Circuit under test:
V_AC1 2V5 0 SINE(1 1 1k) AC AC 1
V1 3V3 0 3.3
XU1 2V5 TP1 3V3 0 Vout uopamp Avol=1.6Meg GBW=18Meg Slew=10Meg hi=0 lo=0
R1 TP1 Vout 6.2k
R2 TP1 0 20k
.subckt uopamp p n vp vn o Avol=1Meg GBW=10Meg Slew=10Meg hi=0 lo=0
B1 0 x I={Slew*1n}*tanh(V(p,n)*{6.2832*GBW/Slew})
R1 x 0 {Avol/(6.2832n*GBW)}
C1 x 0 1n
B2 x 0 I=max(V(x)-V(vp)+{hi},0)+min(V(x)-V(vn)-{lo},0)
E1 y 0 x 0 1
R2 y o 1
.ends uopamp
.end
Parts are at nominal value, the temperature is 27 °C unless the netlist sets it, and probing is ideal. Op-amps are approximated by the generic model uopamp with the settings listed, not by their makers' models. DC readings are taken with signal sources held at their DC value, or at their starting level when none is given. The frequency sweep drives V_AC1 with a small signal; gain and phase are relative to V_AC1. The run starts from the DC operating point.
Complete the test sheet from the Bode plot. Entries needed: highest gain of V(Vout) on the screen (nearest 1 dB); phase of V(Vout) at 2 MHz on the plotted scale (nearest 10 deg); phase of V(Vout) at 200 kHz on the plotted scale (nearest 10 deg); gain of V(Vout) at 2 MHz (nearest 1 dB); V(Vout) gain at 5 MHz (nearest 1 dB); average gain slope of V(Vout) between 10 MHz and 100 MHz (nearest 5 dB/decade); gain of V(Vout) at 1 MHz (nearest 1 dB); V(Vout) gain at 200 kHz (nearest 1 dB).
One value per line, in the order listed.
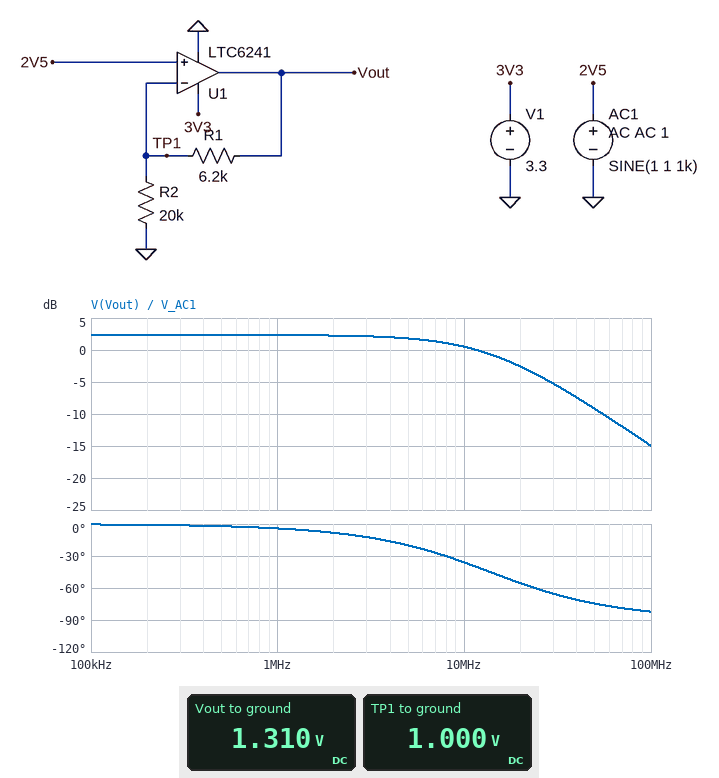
2 dB
-10 deg
0 deg
2 dB
2 dB
-15 dB/decade
2 dB
2 dB
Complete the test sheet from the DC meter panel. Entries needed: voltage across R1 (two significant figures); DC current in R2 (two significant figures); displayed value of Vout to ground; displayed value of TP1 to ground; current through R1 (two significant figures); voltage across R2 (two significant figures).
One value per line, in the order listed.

310 mV
50 µA
1.310 V
1.000 V
50 µA
1.0 V
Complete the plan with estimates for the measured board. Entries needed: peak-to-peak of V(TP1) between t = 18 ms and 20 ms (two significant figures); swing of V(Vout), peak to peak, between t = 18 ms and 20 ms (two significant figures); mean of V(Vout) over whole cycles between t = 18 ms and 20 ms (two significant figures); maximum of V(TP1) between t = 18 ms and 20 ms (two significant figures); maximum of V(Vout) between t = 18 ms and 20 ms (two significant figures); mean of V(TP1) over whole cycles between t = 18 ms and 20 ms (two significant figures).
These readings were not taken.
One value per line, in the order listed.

2.0 V
2.6 V
1.3 V
2.0 V
2.6 V
1.0 V
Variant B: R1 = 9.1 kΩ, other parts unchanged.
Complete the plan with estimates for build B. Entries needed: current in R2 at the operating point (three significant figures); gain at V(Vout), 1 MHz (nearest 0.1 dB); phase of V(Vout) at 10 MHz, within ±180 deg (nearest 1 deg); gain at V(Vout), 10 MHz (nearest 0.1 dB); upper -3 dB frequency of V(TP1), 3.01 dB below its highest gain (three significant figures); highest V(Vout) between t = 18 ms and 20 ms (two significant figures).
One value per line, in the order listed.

50.0 µA
3.2 dB
-39 deg
1.1 dB
12.4 MHz
2.9 V
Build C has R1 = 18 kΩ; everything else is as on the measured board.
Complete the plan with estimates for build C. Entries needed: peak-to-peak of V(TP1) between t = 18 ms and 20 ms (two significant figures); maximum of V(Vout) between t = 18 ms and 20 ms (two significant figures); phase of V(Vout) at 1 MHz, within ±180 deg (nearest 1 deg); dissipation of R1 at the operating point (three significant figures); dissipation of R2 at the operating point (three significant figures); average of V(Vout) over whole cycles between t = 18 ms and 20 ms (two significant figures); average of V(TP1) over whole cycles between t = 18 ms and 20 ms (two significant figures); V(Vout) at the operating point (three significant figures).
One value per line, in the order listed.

1.7 V
3.3 V
-6 deg
45.0 µW
50.0 µW
1.8 V
960 mV
1.90 V
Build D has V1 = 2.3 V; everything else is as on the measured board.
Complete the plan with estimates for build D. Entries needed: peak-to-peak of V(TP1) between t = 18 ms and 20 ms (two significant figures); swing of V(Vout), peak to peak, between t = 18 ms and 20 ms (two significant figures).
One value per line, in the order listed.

1.8 V
2.3 V
